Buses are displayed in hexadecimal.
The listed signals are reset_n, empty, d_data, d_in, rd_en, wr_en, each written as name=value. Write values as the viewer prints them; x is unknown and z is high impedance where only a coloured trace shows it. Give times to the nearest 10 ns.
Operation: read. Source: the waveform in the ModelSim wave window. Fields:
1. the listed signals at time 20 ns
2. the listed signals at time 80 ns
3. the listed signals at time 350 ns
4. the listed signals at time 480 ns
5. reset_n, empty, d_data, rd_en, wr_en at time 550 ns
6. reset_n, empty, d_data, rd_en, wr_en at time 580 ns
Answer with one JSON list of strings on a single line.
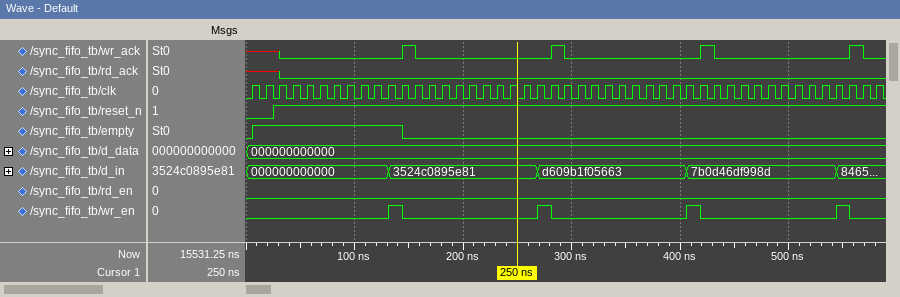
["reset_n=0, empty=1, d_data=000000000000, d_in=000000000000, rd_en=0, wr_en=0", "reset_n=1, empty=1, d_data=000000000000, d_in=000000000000, rd_en=0, wr_en=0", "reset_n=1, empty=0, d_data=000000000000, d_in=d609b1f05663, rd_en=0, wr_en=0", "reset_n=1, empty=0, d_data=000000000000, d_in=7b0d46df998d, rd_en=0, wr_en=0", "reset_n=1, empty=0, d_data=000000000000, rd_en=0, wr_en=1", "reset_n=1, empty=0, d_data=000000000000, rd_en=0, wr_en=0"]
